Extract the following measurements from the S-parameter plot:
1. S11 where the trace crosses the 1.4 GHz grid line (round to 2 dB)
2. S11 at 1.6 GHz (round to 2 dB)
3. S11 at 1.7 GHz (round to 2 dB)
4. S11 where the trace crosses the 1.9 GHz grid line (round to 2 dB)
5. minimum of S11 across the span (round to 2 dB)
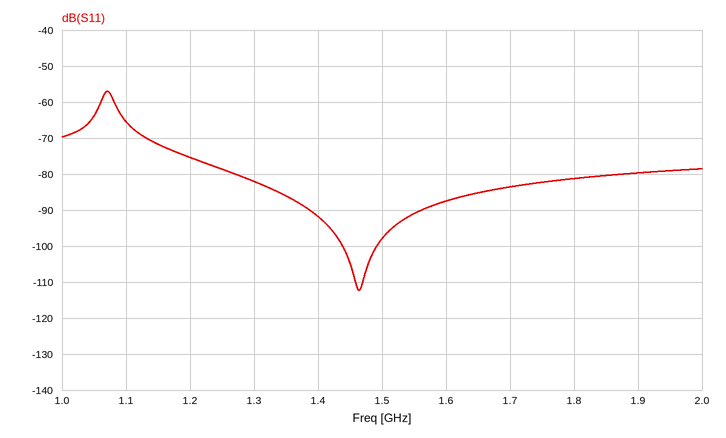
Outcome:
-92 dB
-88 dB
-84 dB
-80 dB
-112 dB
